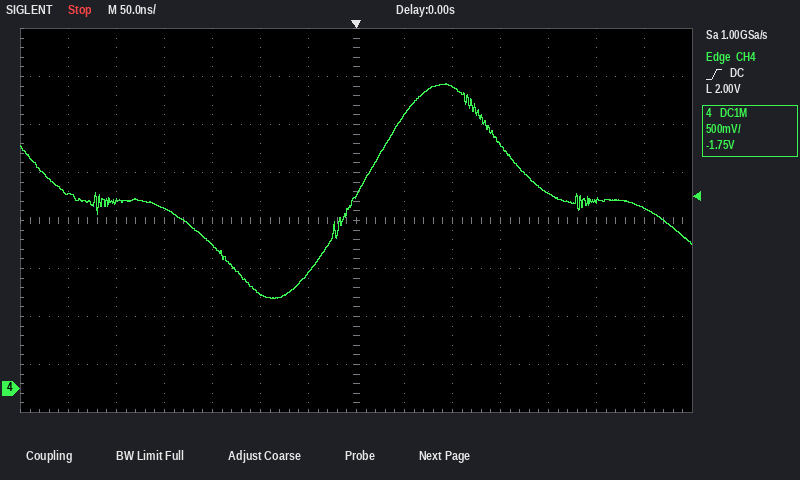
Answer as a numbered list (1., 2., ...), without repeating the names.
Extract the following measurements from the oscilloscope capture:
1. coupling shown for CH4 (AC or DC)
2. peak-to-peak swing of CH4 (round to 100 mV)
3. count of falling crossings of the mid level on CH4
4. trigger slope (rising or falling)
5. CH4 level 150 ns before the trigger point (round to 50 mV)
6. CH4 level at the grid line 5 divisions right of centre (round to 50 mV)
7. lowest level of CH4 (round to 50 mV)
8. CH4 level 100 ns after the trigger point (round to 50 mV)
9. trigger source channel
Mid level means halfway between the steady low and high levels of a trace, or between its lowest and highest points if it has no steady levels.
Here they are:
1. DC
2. 2.20 V
3. 2
4. rising
5. 1.50 V
6. 1.95 V
7. 950 mV
8. 3.15 V
9. CH4
